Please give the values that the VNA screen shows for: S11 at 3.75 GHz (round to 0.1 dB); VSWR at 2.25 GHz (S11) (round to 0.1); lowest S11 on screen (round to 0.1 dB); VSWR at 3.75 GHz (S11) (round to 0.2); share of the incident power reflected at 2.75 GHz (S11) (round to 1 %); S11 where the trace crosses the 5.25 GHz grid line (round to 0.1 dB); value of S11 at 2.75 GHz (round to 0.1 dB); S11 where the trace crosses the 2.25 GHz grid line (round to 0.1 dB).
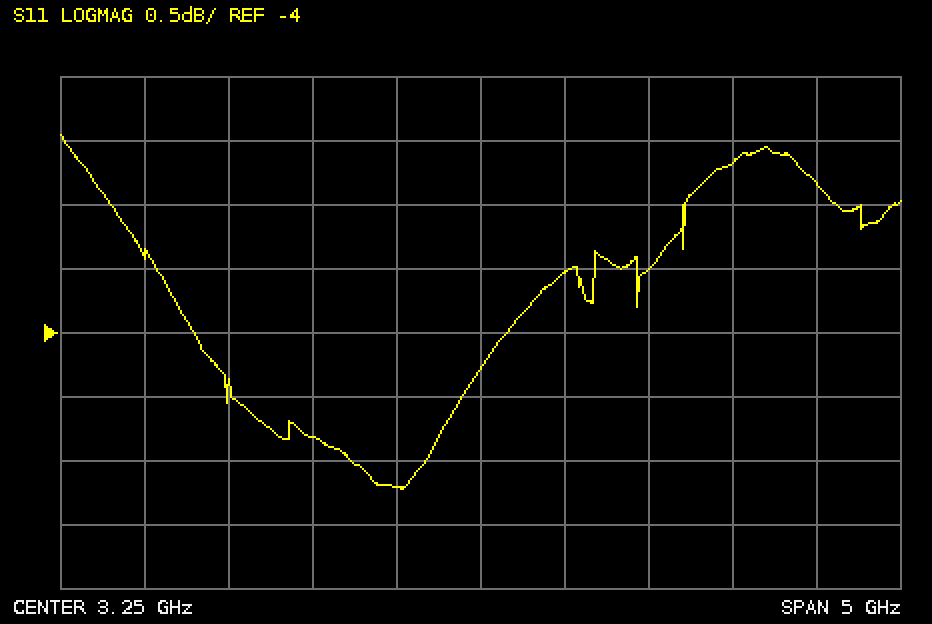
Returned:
-3.5 dB
3.7
-5.2 dB
5.0
30 %
-2.8 dB
-5.2 dB
-4.8 dB
